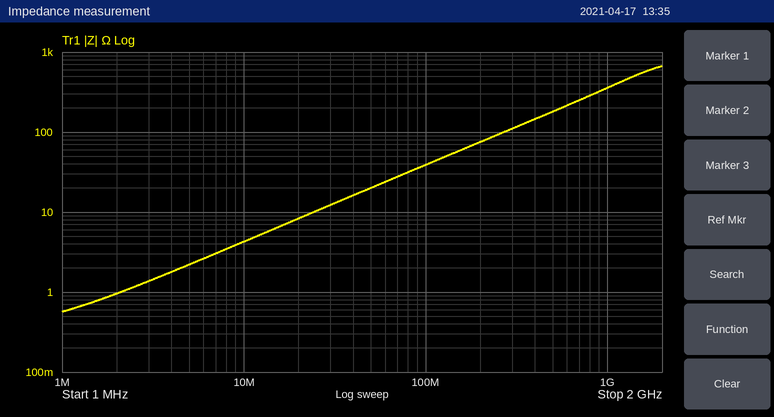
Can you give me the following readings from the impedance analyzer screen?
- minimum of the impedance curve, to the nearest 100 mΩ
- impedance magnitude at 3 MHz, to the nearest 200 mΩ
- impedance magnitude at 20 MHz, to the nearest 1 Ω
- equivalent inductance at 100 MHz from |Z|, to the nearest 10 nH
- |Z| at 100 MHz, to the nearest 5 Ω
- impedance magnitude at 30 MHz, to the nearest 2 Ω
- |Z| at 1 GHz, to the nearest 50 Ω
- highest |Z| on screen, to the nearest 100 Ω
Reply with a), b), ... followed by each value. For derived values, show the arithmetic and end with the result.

a) 600 mΩ
b) 1.4 Ω
c) 8 Ω
d) L = 40 Ω/(2π × 100 MHz) ≈ 63.7 nH, so 60 nH to the nearest 10 nH
e) 40 Ω
f) 12 Ω
g) 350 Ω
h) 700 Ω
